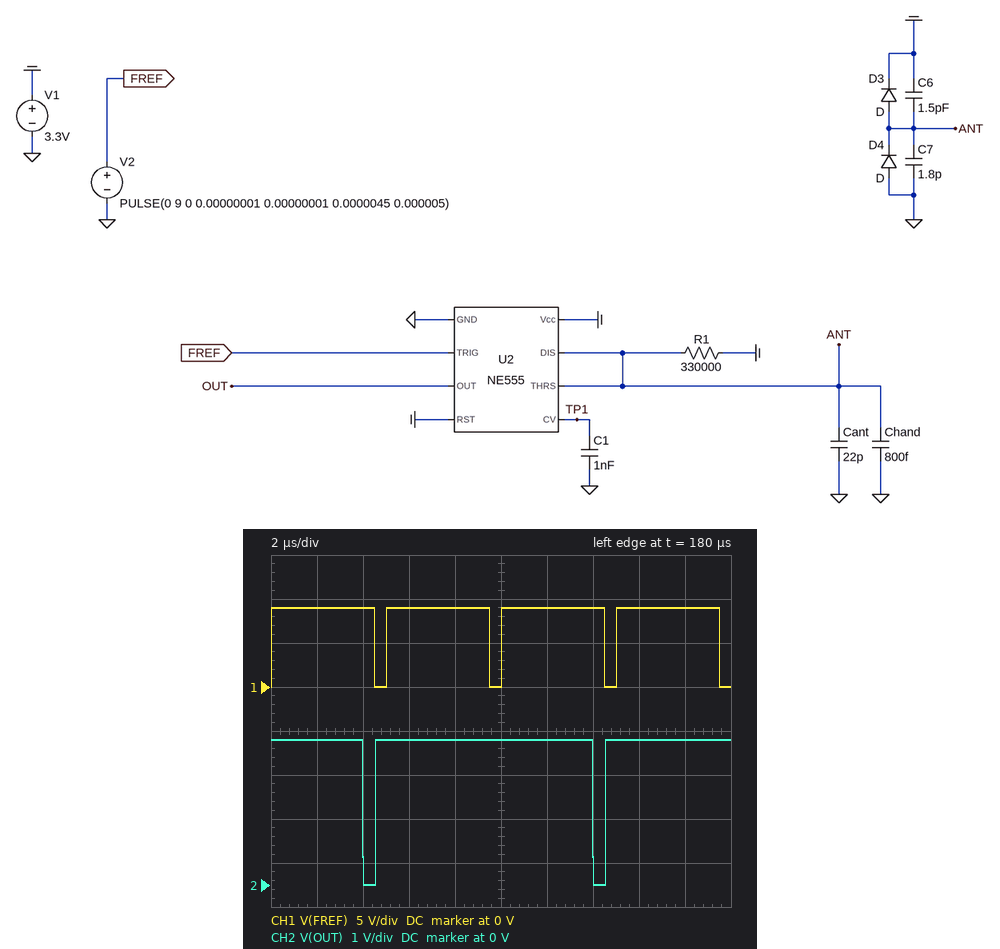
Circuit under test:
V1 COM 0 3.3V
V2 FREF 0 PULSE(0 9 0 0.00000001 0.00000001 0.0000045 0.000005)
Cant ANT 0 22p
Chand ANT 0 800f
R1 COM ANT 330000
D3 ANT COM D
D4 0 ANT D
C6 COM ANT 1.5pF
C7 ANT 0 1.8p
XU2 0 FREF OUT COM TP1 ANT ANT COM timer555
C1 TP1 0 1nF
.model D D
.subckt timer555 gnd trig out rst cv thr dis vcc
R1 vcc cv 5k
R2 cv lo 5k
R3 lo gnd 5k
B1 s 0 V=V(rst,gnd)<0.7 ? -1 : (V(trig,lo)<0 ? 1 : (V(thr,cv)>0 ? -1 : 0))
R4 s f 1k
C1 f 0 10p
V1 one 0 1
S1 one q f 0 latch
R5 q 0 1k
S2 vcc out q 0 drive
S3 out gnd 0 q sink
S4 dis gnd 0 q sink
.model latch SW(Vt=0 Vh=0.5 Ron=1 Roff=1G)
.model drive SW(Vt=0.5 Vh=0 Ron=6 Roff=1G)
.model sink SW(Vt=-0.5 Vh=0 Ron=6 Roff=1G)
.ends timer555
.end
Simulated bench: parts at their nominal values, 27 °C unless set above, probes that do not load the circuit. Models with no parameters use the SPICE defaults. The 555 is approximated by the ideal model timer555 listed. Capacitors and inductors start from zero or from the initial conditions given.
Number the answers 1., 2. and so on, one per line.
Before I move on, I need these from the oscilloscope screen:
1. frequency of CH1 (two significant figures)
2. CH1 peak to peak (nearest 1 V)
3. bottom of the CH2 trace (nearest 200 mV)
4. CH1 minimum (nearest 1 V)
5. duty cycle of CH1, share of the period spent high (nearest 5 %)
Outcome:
1. 200 kHz
2. 9 V
3. 0 V
4. 0 V
5. 90 %
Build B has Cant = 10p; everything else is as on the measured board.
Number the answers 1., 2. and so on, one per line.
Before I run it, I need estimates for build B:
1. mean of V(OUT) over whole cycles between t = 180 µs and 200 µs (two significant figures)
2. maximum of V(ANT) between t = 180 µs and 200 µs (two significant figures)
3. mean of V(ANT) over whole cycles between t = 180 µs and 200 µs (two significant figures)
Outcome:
1. 1.8 V
2. 2.3 V
3. 750 mV
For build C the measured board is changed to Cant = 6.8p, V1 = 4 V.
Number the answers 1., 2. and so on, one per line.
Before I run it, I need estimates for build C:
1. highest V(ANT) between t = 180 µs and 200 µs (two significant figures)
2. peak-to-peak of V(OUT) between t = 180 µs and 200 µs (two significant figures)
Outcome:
1. 2.7 V
2. 4.0 V
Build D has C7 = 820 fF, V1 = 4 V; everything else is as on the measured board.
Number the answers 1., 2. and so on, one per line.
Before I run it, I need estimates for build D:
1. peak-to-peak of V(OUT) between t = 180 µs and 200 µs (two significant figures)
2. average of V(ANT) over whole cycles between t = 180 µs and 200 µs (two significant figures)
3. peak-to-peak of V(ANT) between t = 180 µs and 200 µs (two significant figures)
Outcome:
1. 4.0 V
2. 1.4 V
3. 2.7 V
